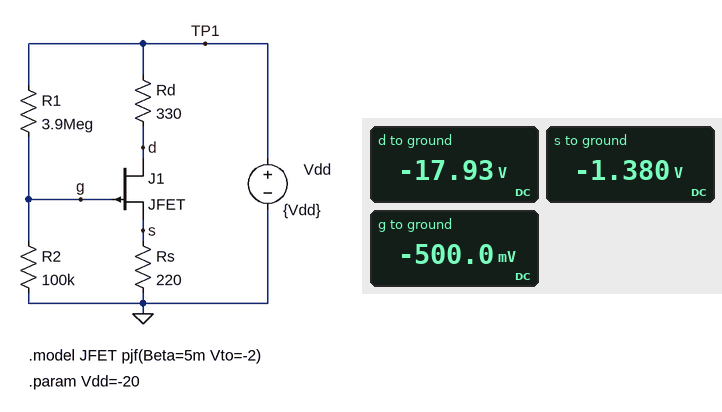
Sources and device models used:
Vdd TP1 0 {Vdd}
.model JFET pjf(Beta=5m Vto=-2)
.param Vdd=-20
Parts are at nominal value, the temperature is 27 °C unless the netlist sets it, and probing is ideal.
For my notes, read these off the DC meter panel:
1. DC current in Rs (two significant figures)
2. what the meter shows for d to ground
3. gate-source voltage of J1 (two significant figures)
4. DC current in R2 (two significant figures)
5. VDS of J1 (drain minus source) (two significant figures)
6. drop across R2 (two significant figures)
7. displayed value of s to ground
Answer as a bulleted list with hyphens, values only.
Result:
- 6.3 mA
- -17.93 V
- 880 mV
- 5.0 µA
- -17 V
- 500 mV
- -1.380 V
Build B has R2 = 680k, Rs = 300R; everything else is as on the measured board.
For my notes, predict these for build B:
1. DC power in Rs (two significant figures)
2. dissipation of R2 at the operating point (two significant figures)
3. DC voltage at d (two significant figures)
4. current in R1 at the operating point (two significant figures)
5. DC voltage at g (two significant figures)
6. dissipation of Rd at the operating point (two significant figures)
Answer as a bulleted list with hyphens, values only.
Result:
- 40 mW
- 13 µW
- -16 V
- 4.4 µA
- -3.0 V
- 44 mW
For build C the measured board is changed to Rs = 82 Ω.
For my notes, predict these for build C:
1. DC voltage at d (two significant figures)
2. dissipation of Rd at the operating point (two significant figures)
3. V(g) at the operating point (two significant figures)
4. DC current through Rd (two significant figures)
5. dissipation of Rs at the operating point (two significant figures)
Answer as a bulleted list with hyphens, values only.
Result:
- -16 V
- 46 mW
- -500 mV
- 12 mA
- 11 mW
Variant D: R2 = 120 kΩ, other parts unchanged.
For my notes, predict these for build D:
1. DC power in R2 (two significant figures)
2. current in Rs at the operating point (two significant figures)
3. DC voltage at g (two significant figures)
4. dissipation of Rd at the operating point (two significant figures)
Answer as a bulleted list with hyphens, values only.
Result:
- 3.0 µW
- 6.6 mA
- -600 mV
- 14 mW
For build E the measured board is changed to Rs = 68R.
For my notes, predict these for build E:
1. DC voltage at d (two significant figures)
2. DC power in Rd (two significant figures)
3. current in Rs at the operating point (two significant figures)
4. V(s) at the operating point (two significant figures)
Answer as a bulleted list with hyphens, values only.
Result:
- -16 V
- 56 mW
- 13 mA
- -890 mV
